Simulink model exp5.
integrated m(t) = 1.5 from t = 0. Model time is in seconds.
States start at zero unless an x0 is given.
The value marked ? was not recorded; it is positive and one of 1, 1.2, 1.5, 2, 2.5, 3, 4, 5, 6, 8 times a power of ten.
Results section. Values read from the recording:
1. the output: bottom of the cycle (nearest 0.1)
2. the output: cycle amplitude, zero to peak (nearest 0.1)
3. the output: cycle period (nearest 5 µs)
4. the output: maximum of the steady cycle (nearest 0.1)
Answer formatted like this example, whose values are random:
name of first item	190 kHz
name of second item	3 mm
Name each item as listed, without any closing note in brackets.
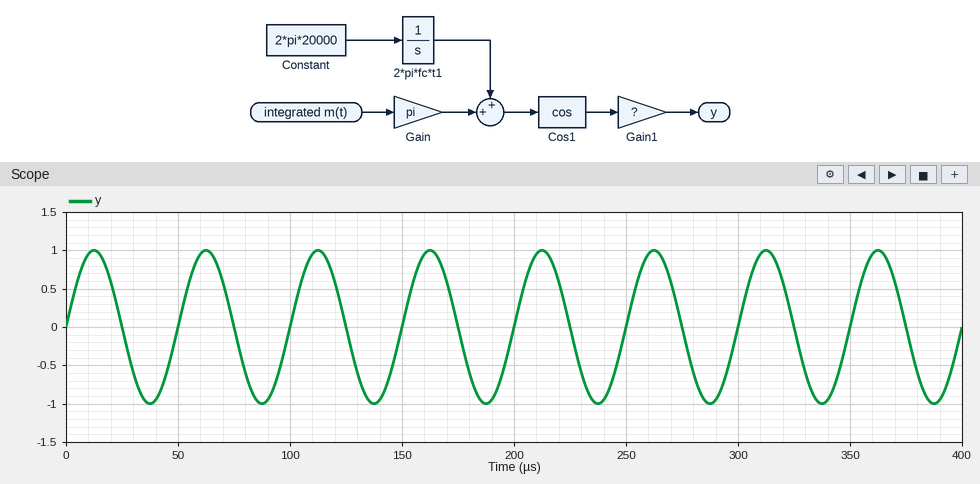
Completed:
the output: bottom of the cycle	-1.0
the output: cycle amplitude, zero to peak	1.0
the output: cycle period	50 µs
the output: maximum of the steady cycle	1.0
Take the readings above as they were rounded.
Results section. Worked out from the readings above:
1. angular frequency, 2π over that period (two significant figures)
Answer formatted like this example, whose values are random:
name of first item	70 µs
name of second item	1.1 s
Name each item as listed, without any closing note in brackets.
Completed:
angular frequency, 2π over that period	0.13 rad/µs
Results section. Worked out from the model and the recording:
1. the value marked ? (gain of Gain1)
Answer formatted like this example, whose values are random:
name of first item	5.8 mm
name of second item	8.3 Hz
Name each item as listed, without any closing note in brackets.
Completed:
the value marked ?	1
